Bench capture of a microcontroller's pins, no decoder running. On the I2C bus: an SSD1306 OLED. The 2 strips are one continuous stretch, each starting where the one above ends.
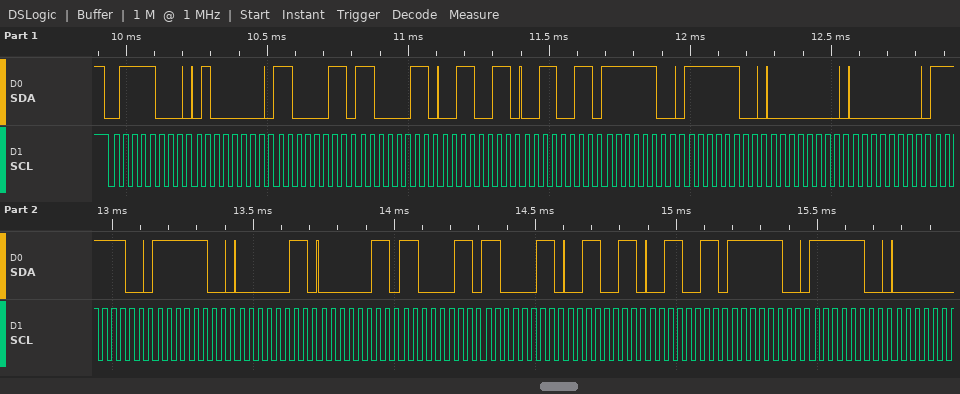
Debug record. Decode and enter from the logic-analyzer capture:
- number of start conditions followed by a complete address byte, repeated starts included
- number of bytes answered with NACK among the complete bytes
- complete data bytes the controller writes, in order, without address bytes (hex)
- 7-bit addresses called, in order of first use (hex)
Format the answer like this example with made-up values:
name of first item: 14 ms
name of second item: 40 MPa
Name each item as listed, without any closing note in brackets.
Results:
number of start conditions followed by a complete address byte, repeated starts included: 1
number of bytes answered with NACK among the complete bytes: 0
complete data bytes the controller writes, in order, without address bytes: 40 C3 C3 33 33 FC FC 00 00 FC FC 03 03 C3 C3 33 33 FC FC
7-bit addresses called, in order of first use: 0x3C
